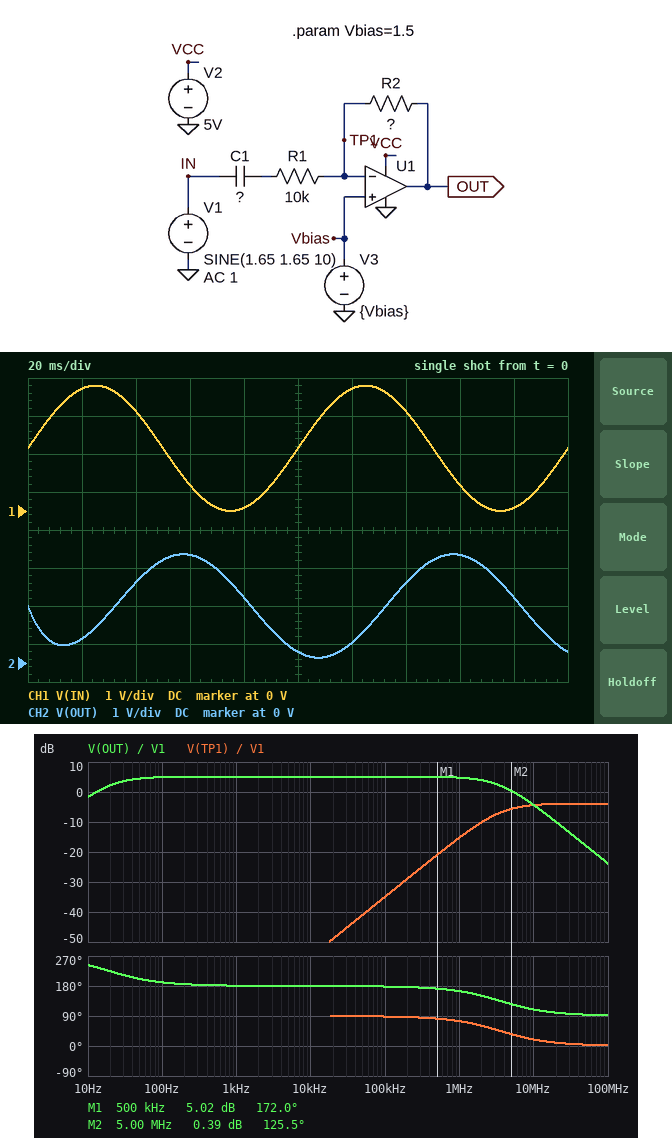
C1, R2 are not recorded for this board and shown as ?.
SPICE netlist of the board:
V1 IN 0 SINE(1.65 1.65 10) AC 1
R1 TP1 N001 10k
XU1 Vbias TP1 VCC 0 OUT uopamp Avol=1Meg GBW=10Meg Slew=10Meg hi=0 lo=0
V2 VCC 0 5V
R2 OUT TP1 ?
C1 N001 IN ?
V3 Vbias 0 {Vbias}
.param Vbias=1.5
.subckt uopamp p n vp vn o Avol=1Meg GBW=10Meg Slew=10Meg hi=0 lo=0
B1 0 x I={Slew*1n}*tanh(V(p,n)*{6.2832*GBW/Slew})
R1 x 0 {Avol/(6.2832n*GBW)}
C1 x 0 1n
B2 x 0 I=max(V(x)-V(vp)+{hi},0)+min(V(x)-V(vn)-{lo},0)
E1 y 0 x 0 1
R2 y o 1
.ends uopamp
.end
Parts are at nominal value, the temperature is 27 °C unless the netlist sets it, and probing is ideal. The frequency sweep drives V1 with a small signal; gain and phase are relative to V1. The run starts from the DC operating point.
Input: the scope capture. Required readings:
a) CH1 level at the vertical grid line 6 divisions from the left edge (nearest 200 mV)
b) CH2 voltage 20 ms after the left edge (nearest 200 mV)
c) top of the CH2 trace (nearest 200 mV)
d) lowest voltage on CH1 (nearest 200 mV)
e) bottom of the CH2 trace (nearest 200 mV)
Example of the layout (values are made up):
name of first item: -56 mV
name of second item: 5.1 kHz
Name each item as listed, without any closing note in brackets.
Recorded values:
CH1 level at the vertical grid line 6 divisions from the left edge: 3.2 V
CH2 voltage 20 ms after the left edge: 600 mV
top of the CH2 trace: 2.8 V
lowest voltage on CH1: 0 V
bottom of the CH2 trace: 200 mV
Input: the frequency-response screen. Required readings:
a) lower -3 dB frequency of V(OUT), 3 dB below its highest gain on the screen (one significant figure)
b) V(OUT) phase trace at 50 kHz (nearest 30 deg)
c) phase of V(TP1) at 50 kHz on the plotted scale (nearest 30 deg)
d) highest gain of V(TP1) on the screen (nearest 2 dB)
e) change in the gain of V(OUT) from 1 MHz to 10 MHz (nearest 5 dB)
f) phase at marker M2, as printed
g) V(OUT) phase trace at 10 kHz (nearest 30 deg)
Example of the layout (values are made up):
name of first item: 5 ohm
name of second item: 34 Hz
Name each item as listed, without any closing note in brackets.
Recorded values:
lower -3 dB frequency of V(OUT), 3 dB below its highest gain on the screen: 20 Hz
V(OUT) phase trace at 50 kHz: 180 deg
phase of V(TP1) at 50 kHz on the plotted scale: 90 deg
highest gain of V(TP1) on the screen: -4 dB
change in the gain of V(OUT) from 1 MHz to 10 MHz: -10 dB
phase at marker M2, as printed: 125.5 deg
V(OUT) phase trace at 10 kHz: 180 deg
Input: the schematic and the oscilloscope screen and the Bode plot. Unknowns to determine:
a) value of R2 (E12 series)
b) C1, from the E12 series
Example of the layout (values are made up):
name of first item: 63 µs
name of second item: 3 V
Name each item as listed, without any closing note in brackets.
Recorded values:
value of R2: 18 kΩ
C1, from the E12 series: 820 nF
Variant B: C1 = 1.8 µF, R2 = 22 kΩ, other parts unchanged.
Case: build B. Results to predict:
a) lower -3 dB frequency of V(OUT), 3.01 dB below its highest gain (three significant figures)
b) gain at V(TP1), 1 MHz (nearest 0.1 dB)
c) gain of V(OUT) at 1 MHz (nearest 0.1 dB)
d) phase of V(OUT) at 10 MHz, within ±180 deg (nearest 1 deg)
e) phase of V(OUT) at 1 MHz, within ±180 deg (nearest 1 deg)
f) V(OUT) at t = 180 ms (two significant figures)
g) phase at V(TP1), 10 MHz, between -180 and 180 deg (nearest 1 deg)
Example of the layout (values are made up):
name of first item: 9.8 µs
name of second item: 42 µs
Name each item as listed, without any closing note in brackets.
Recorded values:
lower -3 dB frequency of V(OUT), 3.01 dB below its highest gain: 8.84 Hz
gain at V(TP1), 1 MHz: -13.6 dB
gain of V(OUT) at 1 MHz: 6.4 dB
phase of V(OUT) at 10 MHz, within ±180 deg: 107 deg
phase of V(OUT) at 1 MHz, within ±180 deg: 162 deg
V(OUT) at t = 180 ms: 2.8 V
phase at V(TP1), 10 MHz, between -180 and 180 deg: 17 deg
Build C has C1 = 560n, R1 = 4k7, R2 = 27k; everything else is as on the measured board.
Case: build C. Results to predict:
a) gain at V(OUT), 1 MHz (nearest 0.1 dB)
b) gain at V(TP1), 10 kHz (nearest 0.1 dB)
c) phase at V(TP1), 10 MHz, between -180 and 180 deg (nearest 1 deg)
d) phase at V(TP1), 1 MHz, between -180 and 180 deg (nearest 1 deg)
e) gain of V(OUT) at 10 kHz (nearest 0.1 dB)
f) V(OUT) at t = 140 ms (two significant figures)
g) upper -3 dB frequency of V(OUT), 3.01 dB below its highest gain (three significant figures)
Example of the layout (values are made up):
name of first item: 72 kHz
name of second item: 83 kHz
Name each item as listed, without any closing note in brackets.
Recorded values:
gain at V(OUT), 1 MHz: 13.6 dB
gain at V(TP1), 10 kHz: -44.8 dB
phase at V(TP1), 10 MHz, between -180 and 180 deg: 8 deg
phase at V(TP1), 1 MHz, between -180 and 180 deg: 56 deg
gain of V(OUT) at 10 kHz: 15.2 dB
V(OUT) at t = 140 ms: 2.6 V
upper -3 dB frequency of V(OUT), 3.01 dB below its highest gain: 1.48 MHz
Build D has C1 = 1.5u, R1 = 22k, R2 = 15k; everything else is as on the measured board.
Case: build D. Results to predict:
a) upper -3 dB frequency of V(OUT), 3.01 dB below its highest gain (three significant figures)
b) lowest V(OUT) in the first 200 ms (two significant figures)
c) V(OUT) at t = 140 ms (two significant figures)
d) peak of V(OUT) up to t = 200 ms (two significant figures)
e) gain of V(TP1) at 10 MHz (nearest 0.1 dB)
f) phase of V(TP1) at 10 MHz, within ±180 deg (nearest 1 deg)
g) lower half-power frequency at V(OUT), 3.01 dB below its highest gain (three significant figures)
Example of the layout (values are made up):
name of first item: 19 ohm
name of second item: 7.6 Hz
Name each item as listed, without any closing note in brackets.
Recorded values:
upper -3 dB frequency of V(OUT), 3.01 dB below its highest gain: 5.95 MHz
lowest V(OUT) in the first 200 ms: 500 mV
V(OUT) at t = 140 ms: 1.3 V
peak of V(OUT) up to t = 200 ms: 2.6 V
gain of V(TP1) at 10 MHz: -9.2 dB
phase of V(TP1) at 10 MHz, within ±180 deg: 31 deg
lower half-power frequency at V(OUT), 3.01 dB below its highest gain: 4.82 Hz
